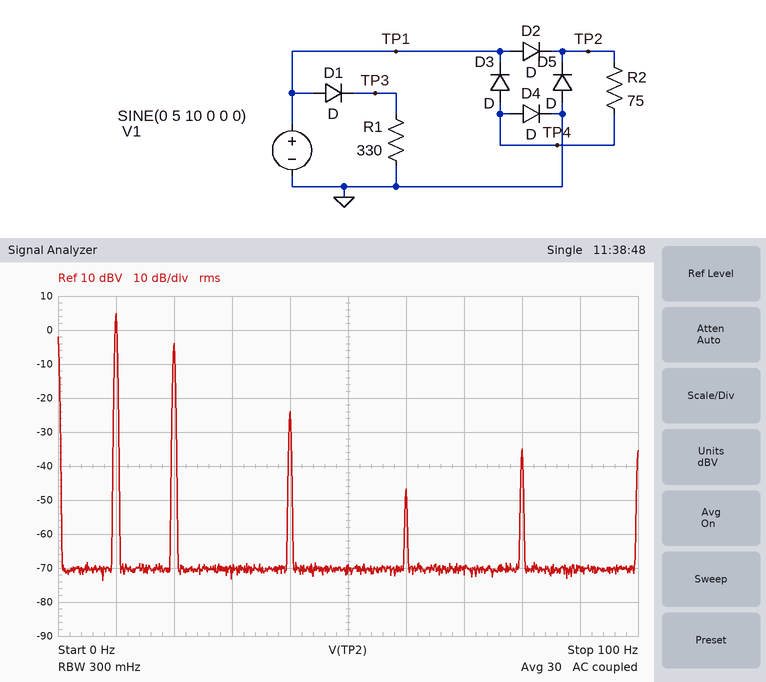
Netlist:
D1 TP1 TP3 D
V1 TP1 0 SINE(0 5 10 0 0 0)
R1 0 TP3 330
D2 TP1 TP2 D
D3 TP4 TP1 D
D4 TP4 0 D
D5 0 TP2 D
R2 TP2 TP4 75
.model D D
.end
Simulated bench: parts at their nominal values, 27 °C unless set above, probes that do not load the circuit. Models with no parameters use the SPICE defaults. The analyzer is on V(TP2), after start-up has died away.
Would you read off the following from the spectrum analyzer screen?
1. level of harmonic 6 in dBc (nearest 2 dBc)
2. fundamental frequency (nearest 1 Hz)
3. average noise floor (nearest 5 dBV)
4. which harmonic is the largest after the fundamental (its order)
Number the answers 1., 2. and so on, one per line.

1. -52 dBc
2. 10 Hz
3. -70 dBV
4. 2
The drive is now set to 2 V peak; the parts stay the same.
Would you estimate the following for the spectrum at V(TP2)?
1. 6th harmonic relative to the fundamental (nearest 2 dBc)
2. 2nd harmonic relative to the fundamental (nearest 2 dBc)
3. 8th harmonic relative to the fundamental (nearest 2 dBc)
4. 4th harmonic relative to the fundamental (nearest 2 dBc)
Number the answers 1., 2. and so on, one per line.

1. -40 dBc
2. -16 dBc
3. -42 dBc
4. -26 dBc
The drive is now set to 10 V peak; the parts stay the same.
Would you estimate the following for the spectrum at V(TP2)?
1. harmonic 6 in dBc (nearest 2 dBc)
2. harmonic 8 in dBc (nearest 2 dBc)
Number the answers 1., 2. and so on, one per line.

1. -32 dBc
2. -42 dBc
